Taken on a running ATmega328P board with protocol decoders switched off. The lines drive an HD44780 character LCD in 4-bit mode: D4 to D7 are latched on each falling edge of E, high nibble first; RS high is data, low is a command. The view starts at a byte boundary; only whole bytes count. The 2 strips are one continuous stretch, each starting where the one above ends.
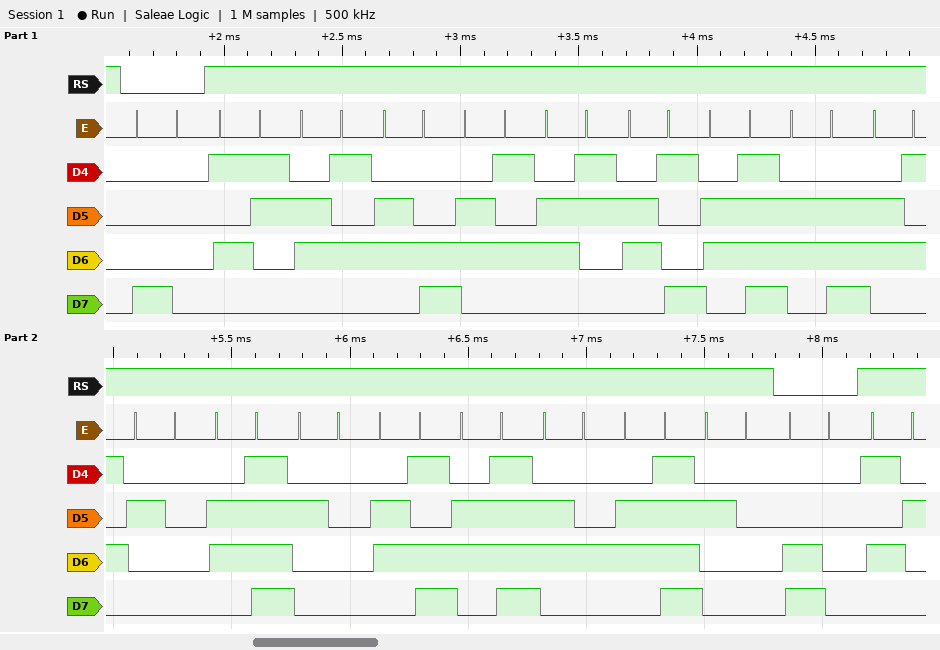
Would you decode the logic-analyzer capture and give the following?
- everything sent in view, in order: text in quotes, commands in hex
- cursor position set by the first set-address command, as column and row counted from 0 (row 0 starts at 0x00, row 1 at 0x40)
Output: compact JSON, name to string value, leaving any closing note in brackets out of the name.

{"everything sent in view, in order: text in quotes, commands in hex": "0x80 \"Selecione o modo \" 0xC0 \"R\"", "cursor position set by the first set-address command, as column and row counted from 0": "column 0, row 0"}
